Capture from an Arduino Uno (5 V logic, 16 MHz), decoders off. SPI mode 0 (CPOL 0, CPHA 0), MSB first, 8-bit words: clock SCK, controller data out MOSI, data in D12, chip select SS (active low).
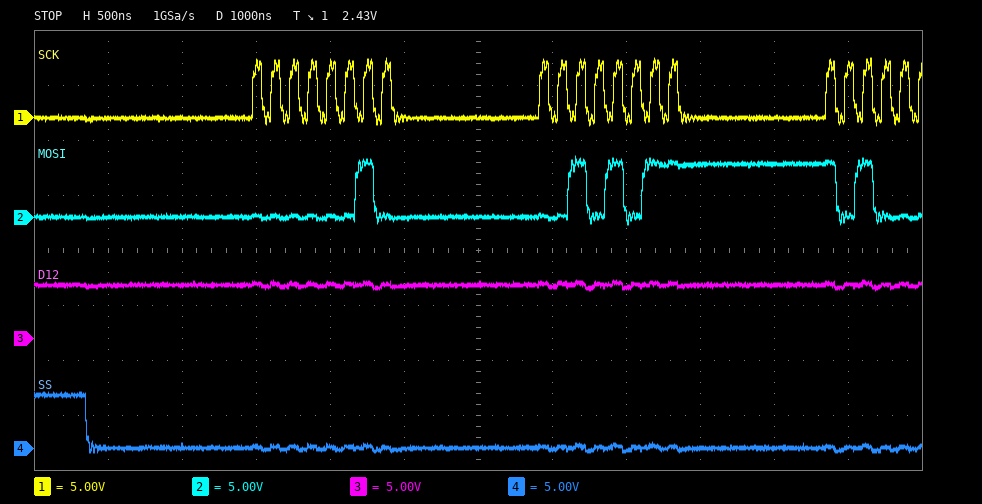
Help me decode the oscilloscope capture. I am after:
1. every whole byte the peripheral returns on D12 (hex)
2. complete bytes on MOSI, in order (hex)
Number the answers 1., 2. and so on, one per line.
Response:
1. FF FF
2. 02 2B
